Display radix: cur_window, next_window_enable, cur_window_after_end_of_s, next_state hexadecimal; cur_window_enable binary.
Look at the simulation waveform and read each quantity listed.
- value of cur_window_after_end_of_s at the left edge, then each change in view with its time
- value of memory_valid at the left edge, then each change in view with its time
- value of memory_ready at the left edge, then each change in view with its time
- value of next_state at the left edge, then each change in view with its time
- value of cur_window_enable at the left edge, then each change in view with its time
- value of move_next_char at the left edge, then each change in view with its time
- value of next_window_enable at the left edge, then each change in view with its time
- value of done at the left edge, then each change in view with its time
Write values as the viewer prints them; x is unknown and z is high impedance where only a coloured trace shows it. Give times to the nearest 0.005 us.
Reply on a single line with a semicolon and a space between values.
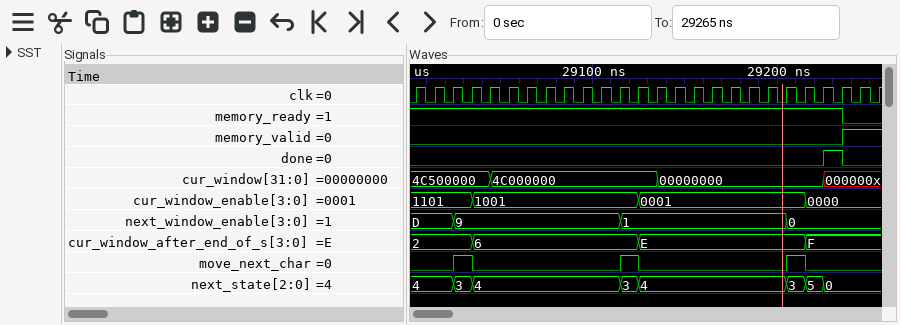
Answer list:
2, 6 at 29.035 us, E at 29.125 us, F at 29.215 us; 0, 1 at 29.235 us; 1, 0 at 29.235 us; 4, 3 at 29.025 us, 4 at 29.035 us, 3 at 29.115 us, 4 at 29.125 us, 3 at 29.205 us, 5 at 29.215 us, 0 at 29.225 us; 1101, 1001 at 29.035 us, 0001 at 29.125 us, 0000 at 29.215 us; 0, 1 at 29.025 us, 0 at 29.035 us, 1 at 29.115 us, 0 at 29.125 us, 1 at 29.205 us, 0 at 29.215 us; D, 9 at 29.025 us, 1 at 29.115 us, 0 at 29.205 us; 0, 1 at 29.225 us, 0 at 29.235 us
